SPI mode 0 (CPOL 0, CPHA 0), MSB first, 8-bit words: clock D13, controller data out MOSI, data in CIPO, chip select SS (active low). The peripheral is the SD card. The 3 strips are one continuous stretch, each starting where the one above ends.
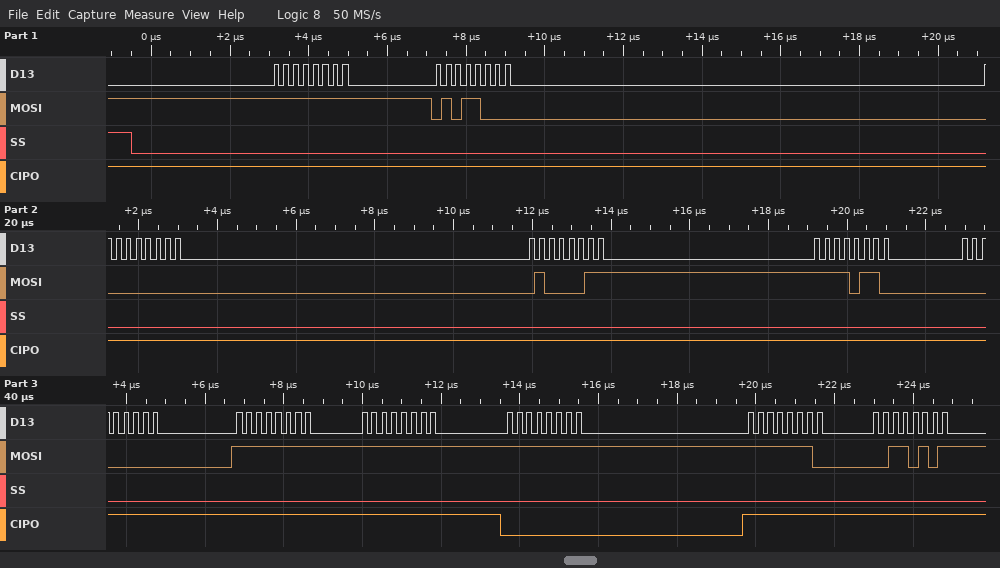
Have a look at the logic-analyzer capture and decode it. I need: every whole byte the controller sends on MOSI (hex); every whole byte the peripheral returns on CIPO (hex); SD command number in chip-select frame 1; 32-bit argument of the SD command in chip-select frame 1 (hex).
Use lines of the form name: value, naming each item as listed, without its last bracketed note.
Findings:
every whole byte the controller sends on MOSI: FF 58 00 43 F6 00 FF FF FF FE 35
every whole byte the peripheral returns on CIPO: FF FF FF FF FF FF FF FF 00 FF FF
SD command number in chip-select frame 1: CMD24
32-bit argument of the SD command in chip-select frame 1: 0x0043F600
